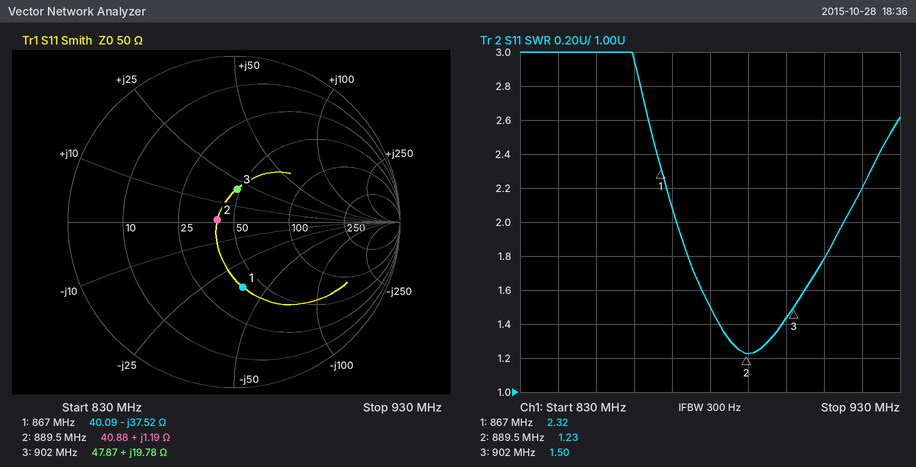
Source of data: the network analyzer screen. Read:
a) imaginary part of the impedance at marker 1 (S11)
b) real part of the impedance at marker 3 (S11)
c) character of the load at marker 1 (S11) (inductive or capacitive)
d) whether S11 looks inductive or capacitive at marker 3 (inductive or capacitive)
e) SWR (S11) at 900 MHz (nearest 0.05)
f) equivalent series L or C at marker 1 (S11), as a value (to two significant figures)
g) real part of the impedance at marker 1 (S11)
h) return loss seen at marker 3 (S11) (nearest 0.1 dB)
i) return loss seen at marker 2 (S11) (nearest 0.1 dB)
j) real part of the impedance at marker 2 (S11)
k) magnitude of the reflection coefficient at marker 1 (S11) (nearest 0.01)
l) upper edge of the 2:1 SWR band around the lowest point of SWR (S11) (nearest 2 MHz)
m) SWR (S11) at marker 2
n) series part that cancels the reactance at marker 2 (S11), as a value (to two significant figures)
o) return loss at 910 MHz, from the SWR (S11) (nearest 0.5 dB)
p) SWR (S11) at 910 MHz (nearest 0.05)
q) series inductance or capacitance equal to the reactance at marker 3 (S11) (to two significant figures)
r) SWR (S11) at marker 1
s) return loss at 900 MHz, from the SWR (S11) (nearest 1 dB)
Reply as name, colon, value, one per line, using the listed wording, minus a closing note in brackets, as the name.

imaginary part of the impedance at marker 1: -37.52 Ω
real part of the impedance at marker 3: 47.87 Ω
character of the load at marker 1 (S11): capacitive
whether S11 looks inductive or capacitive at marker 3: inductive
SWR (S11) at 900 MHz: 1.45
equivalent series L or C at marker 1 (S11), as a value: 4.9 pF
real part of the impedance at marker 1: 40.09 Ω
return loss seen at marker 3 (S11): 14.0 dB
return loss seen at marker 2 (S11): 19.9 dB
real part of the impedance at marker 2: 40.88 Ω
magnitude of the reflection coefficient at marker 1 (S11): 0.40
upper edge of the 2:1 SWR band around the lowest point of SWR (S11): 916 MHz
SWR (S11) at marker 2: 1.23
series part that cancels the reactance at marker 2 (S11), as a value: 150 pF
return loss at 910 MHz, from the SWR (S11): 11.0 dB
SWR (S11) at 910 MHz: 1.80
series inductance or capacitance equal to the reactance at marker 3 (S11): 3.5 nH
SWR (S11) at marker 1: 2.32
return loss at 900 MHz, from the SWR (S11): 15 dB
